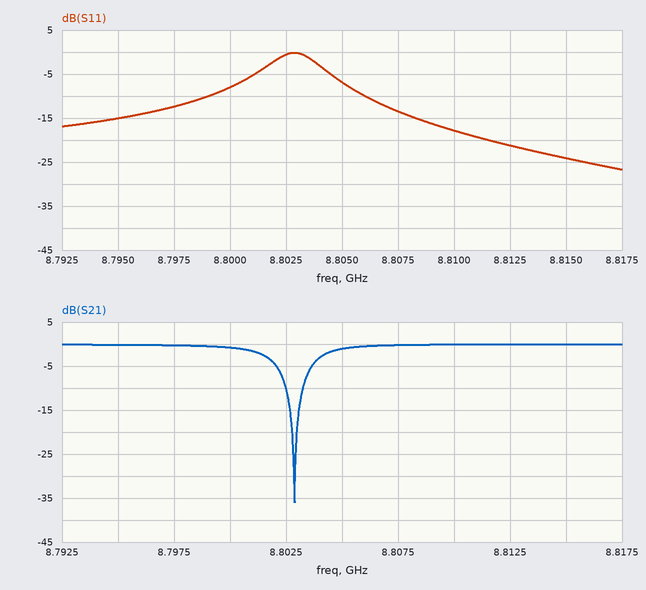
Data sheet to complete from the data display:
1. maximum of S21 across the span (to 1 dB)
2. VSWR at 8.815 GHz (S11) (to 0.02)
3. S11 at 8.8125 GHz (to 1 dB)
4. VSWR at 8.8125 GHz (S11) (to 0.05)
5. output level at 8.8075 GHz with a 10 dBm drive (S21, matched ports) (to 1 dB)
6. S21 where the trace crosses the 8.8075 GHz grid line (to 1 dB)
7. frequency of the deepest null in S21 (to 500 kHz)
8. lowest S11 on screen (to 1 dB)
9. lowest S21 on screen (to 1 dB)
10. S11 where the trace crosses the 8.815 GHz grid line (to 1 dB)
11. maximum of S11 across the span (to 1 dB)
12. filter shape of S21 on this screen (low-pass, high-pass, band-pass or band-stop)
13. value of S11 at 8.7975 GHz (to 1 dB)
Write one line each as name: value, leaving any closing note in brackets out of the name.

maximum of S21 across the span: 0 dB
VSWR at 8.815 GHz (S11): 1.14
S11 at 8.8125 GHz: -21 dB
VSWR at 8.8125 GHz (S11): 1.20
output level at 8.8075 GHz with a 10 dBm drive (S21, matched ports): 10 dBm
S21 where the trace crosses the 8.8075 GHz grid line: 0 dB
frequency of the deepest null in S21: 8.8030 GHz
lowest S11 on screen: -27 dB
lowest S21 on screen: -36 dB
S11 where the trace crosses the 8.815 GHz grid line: -24 dB
maximum of S11 across the span: 0 dB
filter shape of S21 on this screen: band-stop
value of S11 at 8.7975 GHz: -12 dB
